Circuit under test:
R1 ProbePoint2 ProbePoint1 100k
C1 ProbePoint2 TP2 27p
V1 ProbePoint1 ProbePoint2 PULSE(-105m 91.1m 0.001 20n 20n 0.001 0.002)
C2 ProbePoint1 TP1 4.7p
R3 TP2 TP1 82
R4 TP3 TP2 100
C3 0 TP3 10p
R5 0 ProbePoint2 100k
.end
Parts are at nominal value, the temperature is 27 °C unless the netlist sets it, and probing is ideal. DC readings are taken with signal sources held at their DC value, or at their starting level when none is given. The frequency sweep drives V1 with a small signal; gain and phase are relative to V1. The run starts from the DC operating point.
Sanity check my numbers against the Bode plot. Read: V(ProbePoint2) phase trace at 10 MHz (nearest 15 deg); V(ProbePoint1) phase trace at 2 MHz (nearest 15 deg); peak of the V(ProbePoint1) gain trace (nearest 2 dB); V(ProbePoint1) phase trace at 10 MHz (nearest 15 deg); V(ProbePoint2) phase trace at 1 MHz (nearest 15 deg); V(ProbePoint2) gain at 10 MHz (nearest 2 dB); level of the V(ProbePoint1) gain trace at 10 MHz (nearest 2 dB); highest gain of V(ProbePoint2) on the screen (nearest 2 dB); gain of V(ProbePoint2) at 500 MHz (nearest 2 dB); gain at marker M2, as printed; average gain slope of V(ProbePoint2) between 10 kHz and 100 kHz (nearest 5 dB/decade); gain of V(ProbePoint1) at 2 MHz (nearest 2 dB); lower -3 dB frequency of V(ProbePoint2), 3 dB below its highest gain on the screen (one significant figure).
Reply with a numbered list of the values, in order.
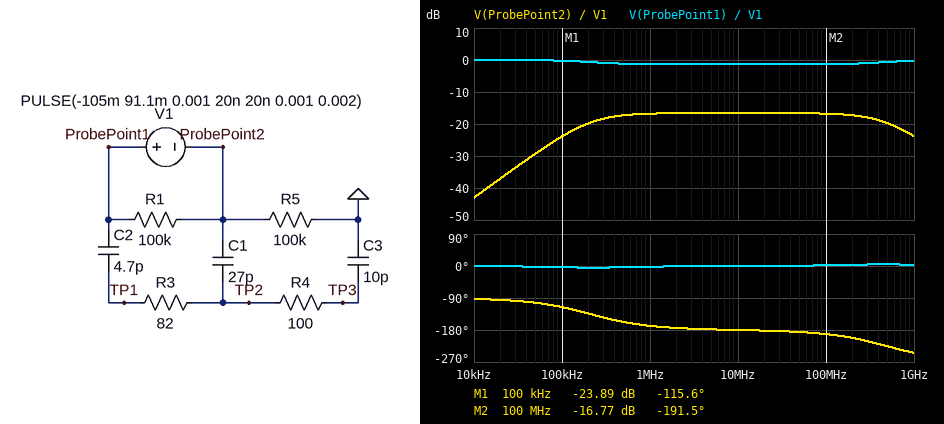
1. -180 deg
2. 0 deg
3. 0 dB
4. 0 deg
5. -165 deg
6. -16 dB
7. -2 dB
8. -16 dB
9. -20 dB
10. -16.77 dB
11. 20 dB/decade
12. -2 dB
13. 200 kHz
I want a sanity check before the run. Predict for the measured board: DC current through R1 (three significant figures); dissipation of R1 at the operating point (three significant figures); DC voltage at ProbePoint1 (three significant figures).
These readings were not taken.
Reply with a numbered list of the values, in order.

1. 1.05 µA
2. 110 nW
3. -105 mV
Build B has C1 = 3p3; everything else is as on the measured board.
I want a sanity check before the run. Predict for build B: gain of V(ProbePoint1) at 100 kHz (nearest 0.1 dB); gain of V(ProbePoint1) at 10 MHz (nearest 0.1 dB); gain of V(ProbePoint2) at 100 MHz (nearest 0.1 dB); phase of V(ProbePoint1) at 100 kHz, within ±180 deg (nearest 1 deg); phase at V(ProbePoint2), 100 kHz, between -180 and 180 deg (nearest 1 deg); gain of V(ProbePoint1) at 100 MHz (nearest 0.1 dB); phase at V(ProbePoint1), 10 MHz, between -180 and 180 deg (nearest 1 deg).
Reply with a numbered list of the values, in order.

1. -0.3 dB
2. -7.7 dB
3. -4.7 dB
4. -9 deg
5. -106 deg
6. -7.5 dB
7. -2 deg
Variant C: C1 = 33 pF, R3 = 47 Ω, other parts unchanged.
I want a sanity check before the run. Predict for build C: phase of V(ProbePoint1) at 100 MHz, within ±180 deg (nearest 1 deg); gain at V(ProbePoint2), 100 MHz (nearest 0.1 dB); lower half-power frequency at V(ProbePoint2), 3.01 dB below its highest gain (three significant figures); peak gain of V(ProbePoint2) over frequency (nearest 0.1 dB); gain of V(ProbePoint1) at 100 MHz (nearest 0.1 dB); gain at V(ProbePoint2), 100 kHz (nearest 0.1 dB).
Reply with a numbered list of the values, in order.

1. 1 deg
2. -18.2 dB
3. 201 kHz
4. -18.1 dB
5. -1.1 dB
6. -25.1 dB
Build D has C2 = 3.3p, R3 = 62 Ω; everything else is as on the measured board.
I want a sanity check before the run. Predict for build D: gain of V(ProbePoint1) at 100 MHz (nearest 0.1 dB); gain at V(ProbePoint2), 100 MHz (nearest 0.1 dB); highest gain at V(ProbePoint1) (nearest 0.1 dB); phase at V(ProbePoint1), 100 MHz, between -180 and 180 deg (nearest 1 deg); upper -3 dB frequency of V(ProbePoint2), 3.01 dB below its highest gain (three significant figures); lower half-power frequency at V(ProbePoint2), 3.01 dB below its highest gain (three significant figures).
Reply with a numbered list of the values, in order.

1. -1.0 dB
2. -19.3 dB
3. 0 dB
4. 1 deg
5. 873 MHz
6. 211 kHz
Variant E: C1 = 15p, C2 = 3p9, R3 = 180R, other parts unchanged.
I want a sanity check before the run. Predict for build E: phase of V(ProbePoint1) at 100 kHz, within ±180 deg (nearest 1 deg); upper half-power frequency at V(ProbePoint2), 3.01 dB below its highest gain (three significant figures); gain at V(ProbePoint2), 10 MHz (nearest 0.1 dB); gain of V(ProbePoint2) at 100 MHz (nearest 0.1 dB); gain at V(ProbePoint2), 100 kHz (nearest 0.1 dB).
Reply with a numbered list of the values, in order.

1. -4 deg
2. 286 MHz
3. -13.7 dB
4. -14.2 dB
5. -22.1 dB
